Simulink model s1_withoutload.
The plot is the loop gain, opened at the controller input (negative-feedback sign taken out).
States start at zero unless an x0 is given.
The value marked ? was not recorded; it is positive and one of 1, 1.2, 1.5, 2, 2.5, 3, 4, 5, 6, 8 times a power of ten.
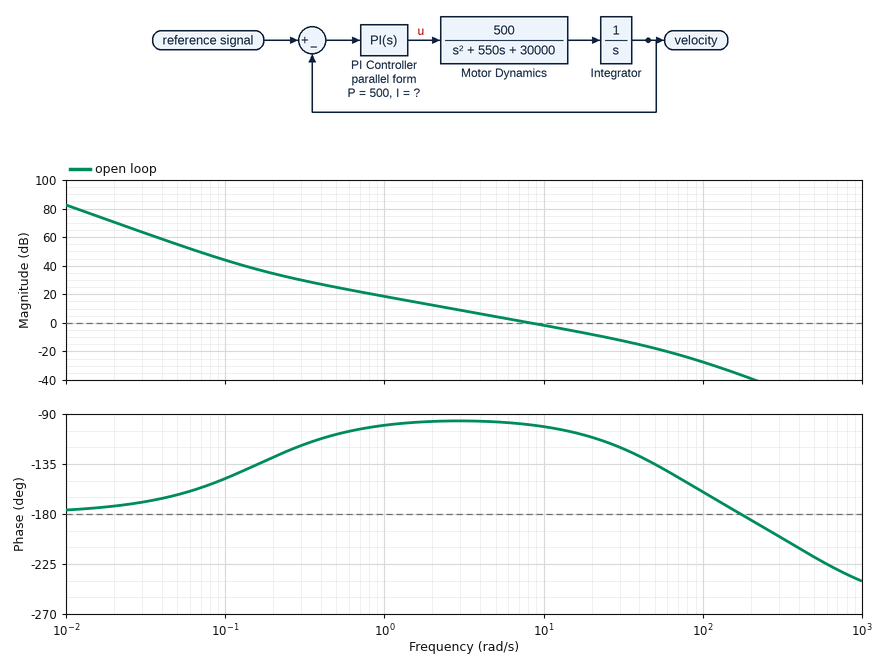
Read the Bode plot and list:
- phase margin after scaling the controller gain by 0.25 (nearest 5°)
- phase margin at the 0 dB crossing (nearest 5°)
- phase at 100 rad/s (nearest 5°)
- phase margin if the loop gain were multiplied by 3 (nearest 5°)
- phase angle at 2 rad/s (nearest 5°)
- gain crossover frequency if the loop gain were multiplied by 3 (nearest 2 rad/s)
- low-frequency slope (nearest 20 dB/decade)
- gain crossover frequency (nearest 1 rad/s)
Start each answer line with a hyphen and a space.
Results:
- 85°
- 80°
- -160°
- 65°
- -95°
- 24 rad/s
- -40 dB/decade
- 8 rad/s
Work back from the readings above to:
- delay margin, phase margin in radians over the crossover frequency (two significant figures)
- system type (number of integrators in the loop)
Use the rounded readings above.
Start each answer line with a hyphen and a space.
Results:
- 0.17 s
- 2
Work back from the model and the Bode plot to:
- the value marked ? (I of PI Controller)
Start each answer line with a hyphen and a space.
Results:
- 80
